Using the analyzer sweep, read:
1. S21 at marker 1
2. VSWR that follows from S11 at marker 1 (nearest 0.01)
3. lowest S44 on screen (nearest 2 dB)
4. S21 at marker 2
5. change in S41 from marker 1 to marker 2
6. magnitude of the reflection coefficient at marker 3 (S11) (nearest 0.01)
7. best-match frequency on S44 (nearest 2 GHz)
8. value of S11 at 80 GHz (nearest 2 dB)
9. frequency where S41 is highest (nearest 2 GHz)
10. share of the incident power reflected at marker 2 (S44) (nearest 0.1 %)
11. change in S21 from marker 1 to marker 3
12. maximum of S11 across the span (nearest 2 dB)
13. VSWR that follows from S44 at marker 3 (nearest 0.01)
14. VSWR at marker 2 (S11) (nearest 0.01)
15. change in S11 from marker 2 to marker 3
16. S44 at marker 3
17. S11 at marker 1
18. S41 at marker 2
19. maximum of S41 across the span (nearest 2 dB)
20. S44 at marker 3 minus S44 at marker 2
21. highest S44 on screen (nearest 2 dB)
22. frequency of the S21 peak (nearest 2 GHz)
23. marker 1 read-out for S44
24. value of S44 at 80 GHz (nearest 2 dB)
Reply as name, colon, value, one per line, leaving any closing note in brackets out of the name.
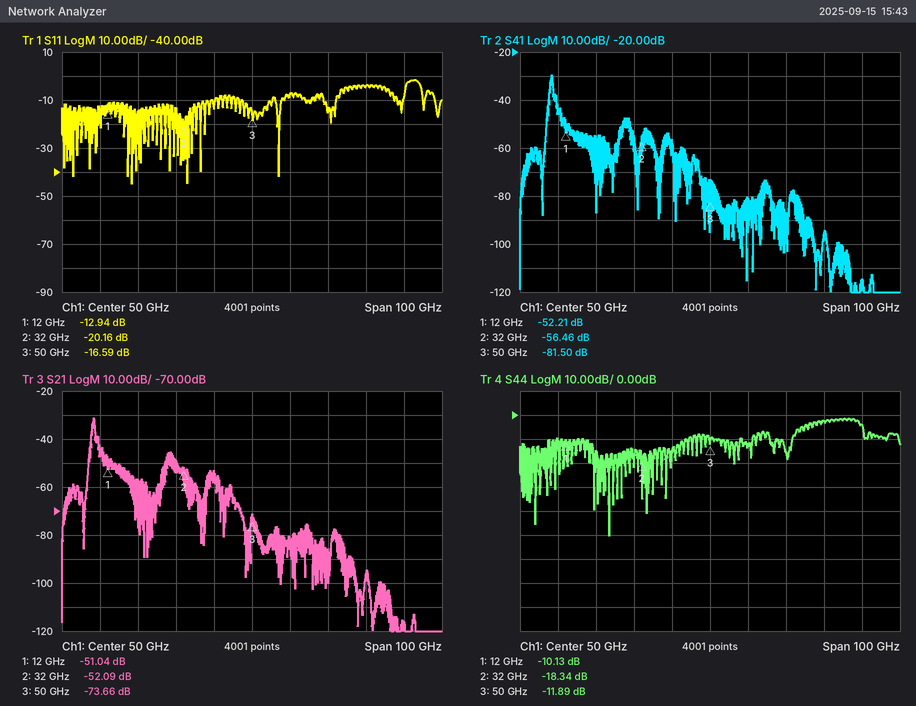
S21 at marker 1: -51.04 dB
VSWR that follows from S11 at marker 1: 1.58
lowest S44 on screen: -50 dB
S21 at marker 2: -52.09 dB
change in S41 from marker 1 to marker 2: -4.25 dB
magnitude of the reflection coefficient at marker 3 (S11): 0.15
best-match frequency on S44: 24 GHz
value of S11 at 80 GHz: -4 dB
frequency where S41 is highest: 8 GHz
share of the incident power reflected at marker 2 (S44): 1.5 %
change in S21 from marker 1 to marker 3: -22.62 dB
maximum of S11 across the span: -2 dB
VSWR that follows from S44 at marker 3: 1.68
VSWR at marker 2 (S11): 1.22
change in S11 from marker 2 to marker 3: 3.57 dB
S44 at marker 3: -11.89 dB
S11 at marker 1: -12.94 dB
S41 at marker 2: -56.46 dB
maximum of S41 across the span: -30 dB
S44 at marker 3 minus S44 at marker 2: 6.45 dB
highest S44 on screen: -2 dB
frequency of the S21 peak: 8 GHz
marker 1 read-out for S44: -10.13 dB
value of S44 at 80 GHz: -2 dB
